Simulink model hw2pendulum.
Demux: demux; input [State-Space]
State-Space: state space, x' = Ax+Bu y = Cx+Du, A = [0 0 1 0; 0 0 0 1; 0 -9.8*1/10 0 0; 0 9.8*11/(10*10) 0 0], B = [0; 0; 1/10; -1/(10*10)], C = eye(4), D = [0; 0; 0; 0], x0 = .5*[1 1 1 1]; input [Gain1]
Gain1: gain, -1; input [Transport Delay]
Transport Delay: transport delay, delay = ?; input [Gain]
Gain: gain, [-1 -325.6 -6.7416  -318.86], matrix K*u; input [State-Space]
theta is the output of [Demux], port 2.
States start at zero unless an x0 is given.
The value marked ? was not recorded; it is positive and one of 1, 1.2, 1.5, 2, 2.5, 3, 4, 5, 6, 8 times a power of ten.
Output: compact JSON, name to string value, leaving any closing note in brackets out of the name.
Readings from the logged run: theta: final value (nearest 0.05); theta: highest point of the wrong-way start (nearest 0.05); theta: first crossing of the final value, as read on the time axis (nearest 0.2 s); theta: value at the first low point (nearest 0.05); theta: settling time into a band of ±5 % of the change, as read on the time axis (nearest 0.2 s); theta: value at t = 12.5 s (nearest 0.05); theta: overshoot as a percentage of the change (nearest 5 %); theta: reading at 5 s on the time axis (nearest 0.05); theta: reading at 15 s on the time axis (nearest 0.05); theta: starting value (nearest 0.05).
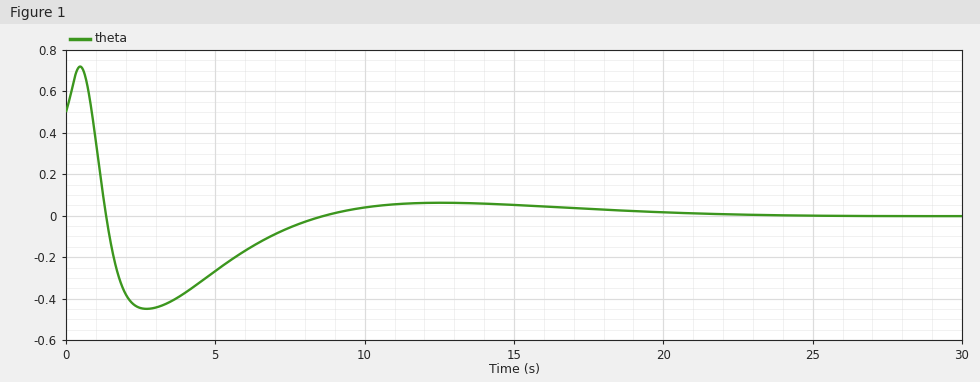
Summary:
{"theta: final value": "0.00", "theta: highest point of the wrong-way start": "0.70", "theta: first crossing of the final value, as read on the time axis": "1.4 s", "theta: value at the first low point": "-0.45", "theta: settling time into a band of ±5 % of the change, as read on the time axis": "18.6 s", "theta: value at t = 12.5 s": "0.05", "theta: overshoot as a percentage of the change": "90 %", "theta: reading at 5 s on the time axis": "-0.25", "theta: reading at 15 s on the time axis": "0.05", "theta: starting value": "0.50"}
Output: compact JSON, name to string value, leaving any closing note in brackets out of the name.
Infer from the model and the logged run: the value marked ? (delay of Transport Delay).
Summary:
{"the value marked ?": "0.25"}
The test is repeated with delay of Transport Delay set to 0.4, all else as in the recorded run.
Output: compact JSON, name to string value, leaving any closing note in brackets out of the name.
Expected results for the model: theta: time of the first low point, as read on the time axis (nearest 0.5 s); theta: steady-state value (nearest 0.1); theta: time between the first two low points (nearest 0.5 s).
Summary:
{"theta: time of the first low point, as read on the time axis": "2.0 s", "theta: steady-state value": "0.0", "theta: time between the first two low points": "2.5 s"}
